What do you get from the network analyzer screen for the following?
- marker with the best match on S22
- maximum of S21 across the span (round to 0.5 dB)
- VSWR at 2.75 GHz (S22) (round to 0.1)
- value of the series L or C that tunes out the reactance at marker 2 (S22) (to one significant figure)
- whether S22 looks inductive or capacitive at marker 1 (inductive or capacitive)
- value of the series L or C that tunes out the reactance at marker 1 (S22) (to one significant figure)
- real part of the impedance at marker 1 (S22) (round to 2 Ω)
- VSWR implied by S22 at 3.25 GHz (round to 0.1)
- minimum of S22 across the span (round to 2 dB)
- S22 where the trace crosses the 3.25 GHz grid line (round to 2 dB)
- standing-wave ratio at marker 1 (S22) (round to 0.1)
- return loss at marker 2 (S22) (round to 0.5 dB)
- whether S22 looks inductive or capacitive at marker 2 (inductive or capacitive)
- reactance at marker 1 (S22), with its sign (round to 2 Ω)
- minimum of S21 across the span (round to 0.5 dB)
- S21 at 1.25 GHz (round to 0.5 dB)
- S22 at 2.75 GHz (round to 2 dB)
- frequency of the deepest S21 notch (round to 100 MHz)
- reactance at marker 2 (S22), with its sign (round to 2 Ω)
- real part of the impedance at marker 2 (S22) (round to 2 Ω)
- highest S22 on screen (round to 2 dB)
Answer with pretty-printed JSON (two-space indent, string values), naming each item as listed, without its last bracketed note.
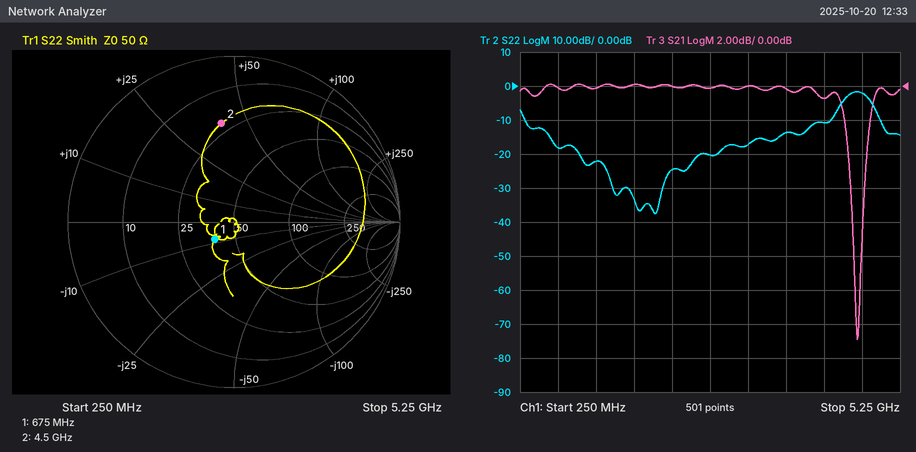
{
  "marker with the best match on S22": "marker 1",
  "maximum of S21 across the span": "0.0 dB",
  "VSWR at 2.75 GHz (S22)": "1.2",
  "value of the series L or C that tunes out the reactance at marker 2 (S22)": "900 fF",
  "whether S22 looks inductive or capacitive at marker 1": "capacitive",
  "value of the series L or C that tunes out the reactance at marker 1 (S22)": "2 nH",
  "real part of the impedance at marker 1 (S22)": "38 Ω",
  "VSWR implied by S22 at 3.25 GHz": "1.3",
  "minimum of S22 across the span": "-38 dB",
  "S22 where the trace crosses the 3.25 GHz grid line": "-18 dB",
  "standing-wave ratio at marker 1 (S22)": "1.4",
  "return loss at marker 2 (S22)": "4.5 dB",
  "whether S22 looks inductive or capacitive at marker 2": "inductive",
  "reactance at marker 1 (S22), with its sign": "-8 Ω",
  "minimum of S21 across the span": "-15.0 dB",
  "S21 at 1.25 GHz": "0.0 dB",
  "S22 at 2.75 GHz": "-20 dB",
  "frequency of the deepest S21 notch": "4.7 GHz",
  "reactance at marker 2 (S22), with its sign": "+40 Ω",
  "real part of the impedance at marker 2 (S22)": "22 Ω",
  "highest S22 on screen": "-2 dB"
}
